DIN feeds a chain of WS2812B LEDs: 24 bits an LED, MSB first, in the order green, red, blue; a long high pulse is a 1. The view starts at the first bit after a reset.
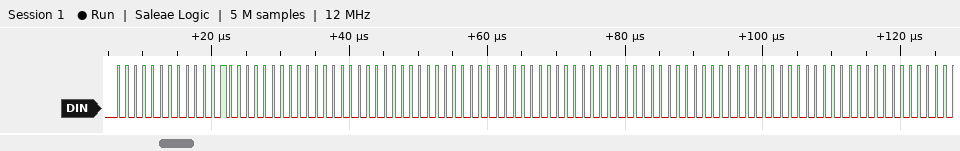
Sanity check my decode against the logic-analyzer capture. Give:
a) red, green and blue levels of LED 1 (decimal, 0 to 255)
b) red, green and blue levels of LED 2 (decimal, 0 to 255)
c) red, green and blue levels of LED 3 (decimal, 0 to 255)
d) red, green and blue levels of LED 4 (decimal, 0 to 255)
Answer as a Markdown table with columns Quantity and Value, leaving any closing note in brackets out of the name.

| Quantity | Value |
|---|---|
| red, green and blue levels of LED 1 | 8, 0, 0 |
| red, green and blue levels of LED 2 | 0, 0, 0 |
| red, green and blue levels of LED 3 | 0, 0, 0 |
| red, green and blue levels of LED 4 | 0, 0, 0 |
